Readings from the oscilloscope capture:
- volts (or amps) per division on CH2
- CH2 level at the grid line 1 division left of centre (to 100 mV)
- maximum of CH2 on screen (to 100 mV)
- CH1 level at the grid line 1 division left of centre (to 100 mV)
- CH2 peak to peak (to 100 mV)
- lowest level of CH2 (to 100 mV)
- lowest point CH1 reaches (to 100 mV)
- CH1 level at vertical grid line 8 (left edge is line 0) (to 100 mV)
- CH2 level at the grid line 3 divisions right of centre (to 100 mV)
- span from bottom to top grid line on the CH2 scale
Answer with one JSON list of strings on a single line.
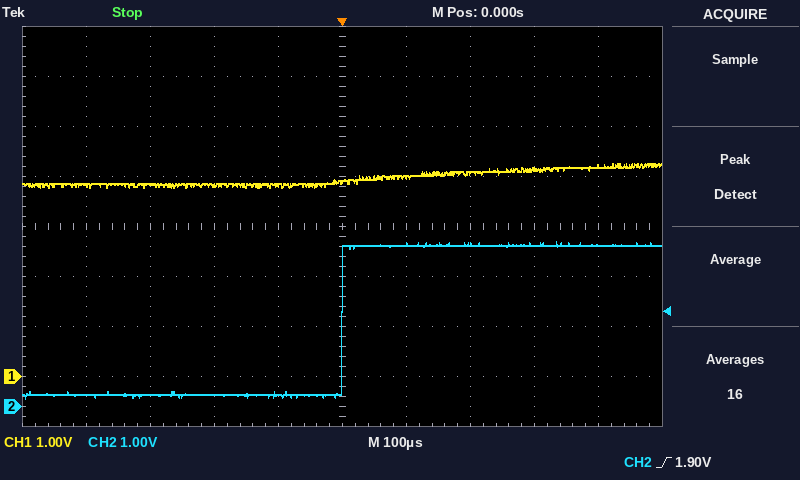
["1 V", "200 mV", "3.3 V", "3.8 V", "3.1 V", "200 mV", "3.8 V", "4.1 V", "3.2 V", "8 V"]
